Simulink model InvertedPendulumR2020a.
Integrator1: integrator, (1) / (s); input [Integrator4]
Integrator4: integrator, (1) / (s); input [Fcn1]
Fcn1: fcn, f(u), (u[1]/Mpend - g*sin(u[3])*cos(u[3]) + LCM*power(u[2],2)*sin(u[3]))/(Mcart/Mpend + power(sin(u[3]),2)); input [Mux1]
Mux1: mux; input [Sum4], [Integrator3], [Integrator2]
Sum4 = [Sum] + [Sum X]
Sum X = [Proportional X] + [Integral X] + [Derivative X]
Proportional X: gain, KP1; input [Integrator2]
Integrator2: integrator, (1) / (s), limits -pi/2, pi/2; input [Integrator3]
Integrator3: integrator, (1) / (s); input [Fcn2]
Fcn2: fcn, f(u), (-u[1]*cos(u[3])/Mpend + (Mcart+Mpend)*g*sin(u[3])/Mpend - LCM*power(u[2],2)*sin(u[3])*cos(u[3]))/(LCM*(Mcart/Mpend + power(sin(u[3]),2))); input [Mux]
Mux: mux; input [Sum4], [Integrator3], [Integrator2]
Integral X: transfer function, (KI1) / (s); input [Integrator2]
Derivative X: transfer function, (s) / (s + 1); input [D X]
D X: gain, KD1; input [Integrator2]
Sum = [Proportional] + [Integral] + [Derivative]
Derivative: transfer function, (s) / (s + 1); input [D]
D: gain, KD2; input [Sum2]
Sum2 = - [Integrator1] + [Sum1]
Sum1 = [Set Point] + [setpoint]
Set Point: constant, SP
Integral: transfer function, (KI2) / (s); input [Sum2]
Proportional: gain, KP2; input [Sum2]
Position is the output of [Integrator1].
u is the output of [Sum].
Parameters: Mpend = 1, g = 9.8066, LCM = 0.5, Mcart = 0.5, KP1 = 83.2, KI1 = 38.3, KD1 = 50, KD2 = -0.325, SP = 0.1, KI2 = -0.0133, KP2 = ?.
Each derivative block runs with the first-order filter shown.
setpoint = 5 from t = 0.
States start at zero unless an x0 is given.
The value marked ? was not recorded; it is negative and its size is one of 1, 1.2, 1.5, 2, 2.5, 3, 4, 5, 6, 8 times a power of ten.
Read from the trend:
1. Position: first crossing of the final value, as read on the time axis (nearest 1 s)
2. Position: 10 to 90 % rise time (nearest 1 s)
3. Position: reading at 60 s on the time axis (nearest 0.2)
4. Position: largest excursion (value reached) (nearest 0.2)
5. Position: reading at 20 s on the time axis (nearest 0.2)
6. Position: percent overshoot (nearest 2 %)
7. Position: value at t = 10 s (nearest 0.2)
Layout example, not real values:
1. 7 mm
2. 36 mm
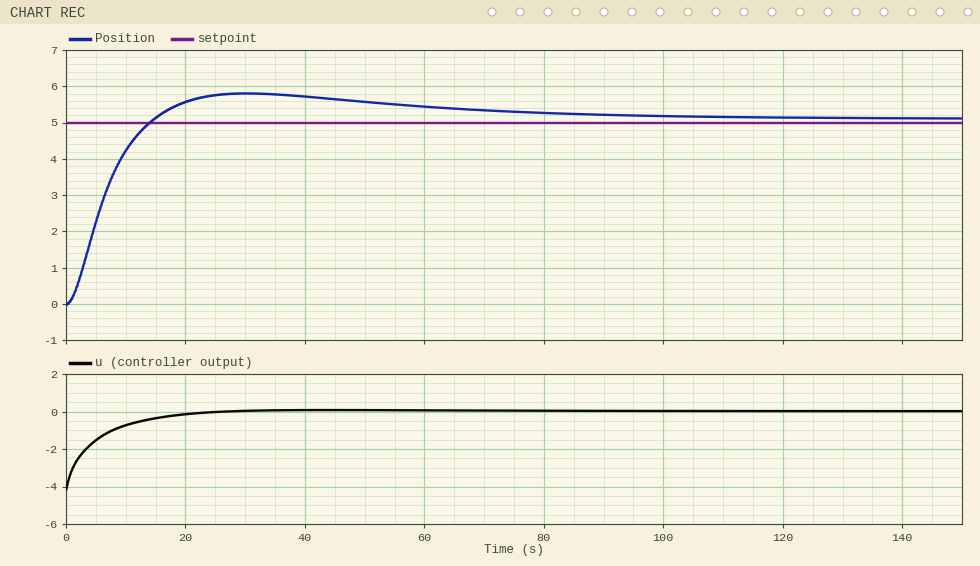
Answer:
1. 15 s
2. 10 s
3. 5.4
4. 5.8
5. 5.6
6. 14 %
7. 4.2
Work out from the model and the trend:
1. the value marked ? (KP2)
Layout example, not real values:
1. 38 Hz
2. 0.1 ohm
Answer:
1. -0.5
